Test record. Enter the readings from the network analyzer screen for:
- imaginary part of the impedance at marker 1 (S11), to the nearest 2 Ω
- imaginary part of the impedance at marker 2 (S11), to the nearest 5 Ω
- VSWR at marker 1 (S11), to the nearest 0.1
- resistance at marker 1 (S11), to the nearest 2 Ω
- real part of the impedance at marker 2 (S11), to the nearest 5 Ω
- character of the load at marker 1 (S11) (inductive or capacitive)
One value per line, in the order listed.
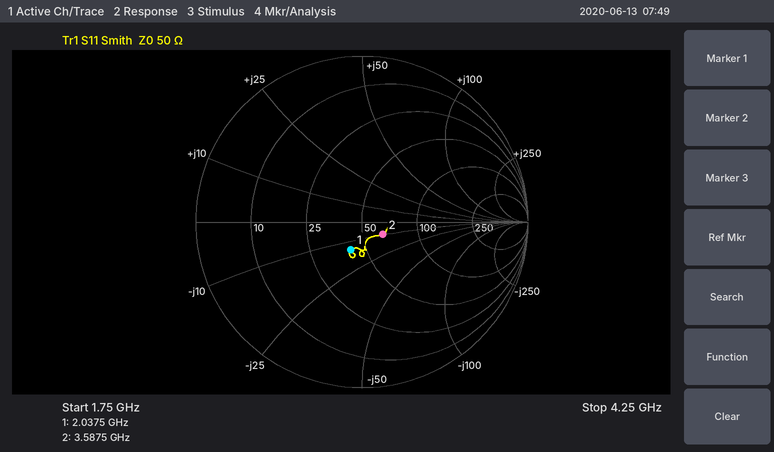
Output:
-14 Ω
-10 Ω
1.4
42 Ω
65 Ω
capacitive
